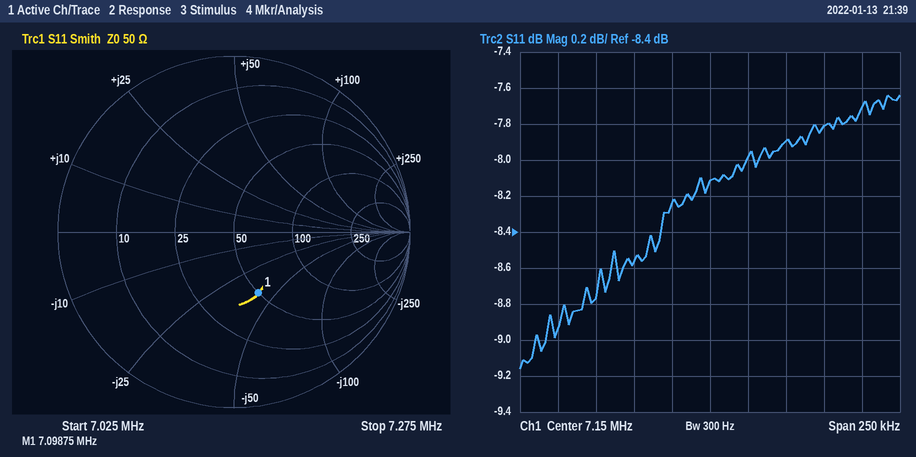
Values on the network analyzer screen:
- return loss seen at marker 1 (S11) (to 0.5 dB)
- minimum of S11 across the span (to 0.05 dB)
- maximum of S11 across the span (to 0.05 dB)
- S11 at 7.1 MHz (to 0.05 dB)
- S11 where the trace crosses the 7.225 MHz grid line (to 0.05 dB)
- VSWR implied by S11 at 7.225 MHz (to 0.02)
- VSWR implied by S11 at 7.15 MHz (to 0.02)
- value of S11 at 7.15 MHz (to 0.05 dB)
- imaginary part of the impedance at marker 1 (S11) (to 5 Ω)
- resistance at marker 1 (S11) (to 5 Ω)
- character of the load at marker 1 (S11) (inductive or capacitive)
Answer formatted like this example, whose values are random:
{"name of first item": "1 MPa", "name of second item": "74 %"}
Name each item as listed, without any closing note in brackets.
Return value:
{"return loss seen at marker 1 (S11)": "8.5 dB", "minimum of S11 across the span": "-9.15 dB", "maximum of S11 across the span": "-7.65 dB", "S11 at 7.1 MHz": "-8.55 dB", "S11 where the trace crosses the 7.225 MHz grid line": "-7.80 dB", "VSWR implied by S11 at 7.225 MHz": "2.38", "VSWR implied by S11 at 7.15 MHz": "2.30", "value of S11 at 7.15 MHz": "-8.10 dB", "imaginary part of the impedance at marker 1 (S11)": "-40 Ω", "resistance at marker 1 (S11)": "50 Ω", "character of the load at marker 1 (S11)": "capacitive"}
